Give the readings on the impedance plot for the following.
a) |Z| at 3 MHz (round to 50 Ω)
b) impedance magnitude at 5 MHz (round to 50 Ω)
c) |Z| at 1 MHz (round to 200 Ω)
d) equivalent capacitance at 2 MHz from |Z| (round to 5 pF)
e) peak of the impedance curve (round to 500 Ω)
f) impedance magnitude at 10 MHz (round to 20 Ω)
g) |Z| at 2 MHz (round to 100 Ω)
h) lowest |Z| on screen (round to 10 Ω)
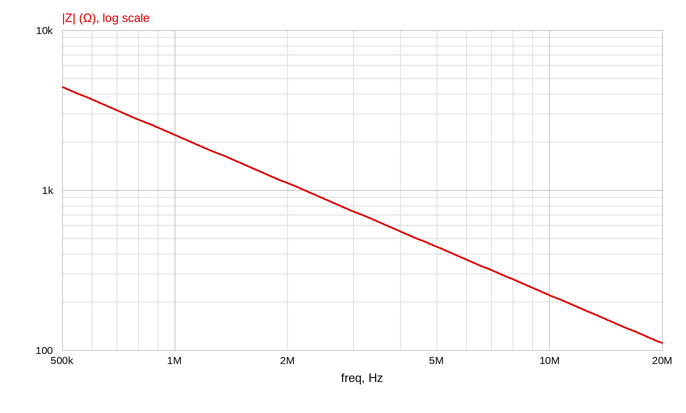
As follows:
750 Ω
450 Ω
2.2 kΩ
70 pF
4.5 kΩ
220 Ω
1.1 kΩ
110 Ω
